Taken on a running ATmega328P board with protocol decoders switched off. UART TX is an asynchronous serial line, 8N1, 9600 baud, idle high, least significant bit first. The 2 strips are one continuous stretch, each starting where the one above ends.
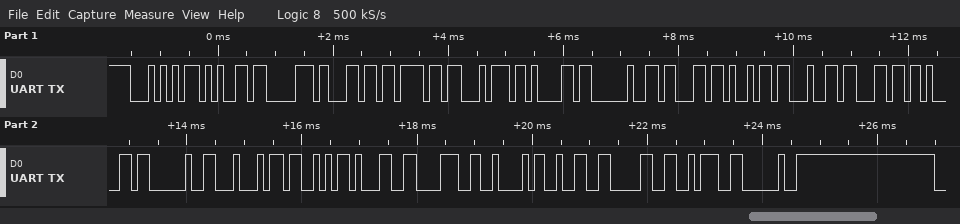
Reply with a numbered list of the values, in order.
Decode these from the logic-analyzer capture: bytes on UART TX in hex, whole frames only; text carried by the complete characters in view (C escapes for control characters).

1. 0x54 0x65 0x70 0x6C 0x6F 0x74 0x61 0x20 0x63 0x69 0x64 0x6C 0x61 0x20 0x44 0x53 0x31 0x38 0x42 0x32 0x30 0x3A 0x20
2. "Teplota cidla DS18B20: "
